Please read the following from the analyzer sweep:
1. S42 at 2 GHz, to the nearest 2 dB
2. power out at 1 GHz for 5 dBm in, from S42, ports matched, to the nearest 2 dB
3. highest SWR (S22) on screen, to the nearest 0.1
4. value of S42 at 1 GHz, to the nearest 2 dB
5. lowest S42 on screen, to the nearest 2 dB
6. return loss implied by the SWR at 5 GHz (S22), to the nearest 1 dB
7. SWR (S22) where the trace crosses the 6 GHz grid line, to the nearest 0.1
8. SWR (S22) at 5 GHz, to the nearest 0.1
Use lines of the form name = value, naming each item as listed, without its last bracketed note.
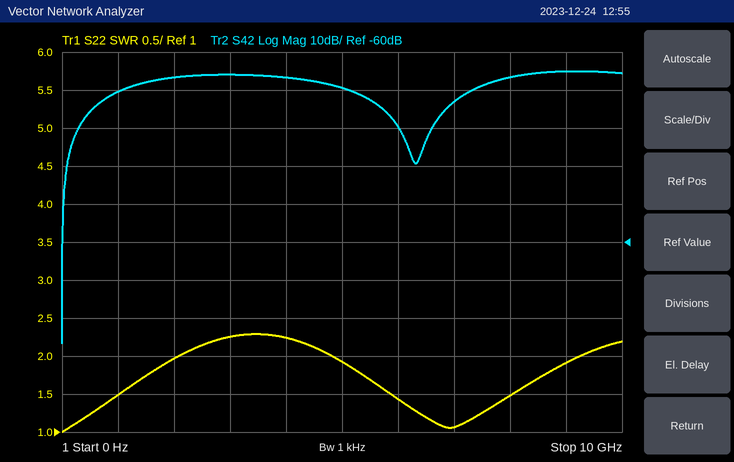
S42 at 2 GHz, to the nearest 2 dB = -16 dB
power out at 1 GHz for 5 dBm in, from S42, ports matched, to the nearest 2 dB = -16 dBm
highest SWR (S22) on screen, to the nearest 0.1 = 2.3
value of S42 at 1 GHz, to the nearest 2 dB = -20 dB
lowest S42 on screen, to the nearest 2 dB = -86 dB
return loss implied by the SWR at 5 GHz (S22), to the nearest 1 dB = 10 dB
SWR (S22) where the trace crosses the 6 GHz grid line, to the nearest 0.1 = 1.4
SWR (S22) at 5 GHz, to the nearest 0.1 = 1.9
